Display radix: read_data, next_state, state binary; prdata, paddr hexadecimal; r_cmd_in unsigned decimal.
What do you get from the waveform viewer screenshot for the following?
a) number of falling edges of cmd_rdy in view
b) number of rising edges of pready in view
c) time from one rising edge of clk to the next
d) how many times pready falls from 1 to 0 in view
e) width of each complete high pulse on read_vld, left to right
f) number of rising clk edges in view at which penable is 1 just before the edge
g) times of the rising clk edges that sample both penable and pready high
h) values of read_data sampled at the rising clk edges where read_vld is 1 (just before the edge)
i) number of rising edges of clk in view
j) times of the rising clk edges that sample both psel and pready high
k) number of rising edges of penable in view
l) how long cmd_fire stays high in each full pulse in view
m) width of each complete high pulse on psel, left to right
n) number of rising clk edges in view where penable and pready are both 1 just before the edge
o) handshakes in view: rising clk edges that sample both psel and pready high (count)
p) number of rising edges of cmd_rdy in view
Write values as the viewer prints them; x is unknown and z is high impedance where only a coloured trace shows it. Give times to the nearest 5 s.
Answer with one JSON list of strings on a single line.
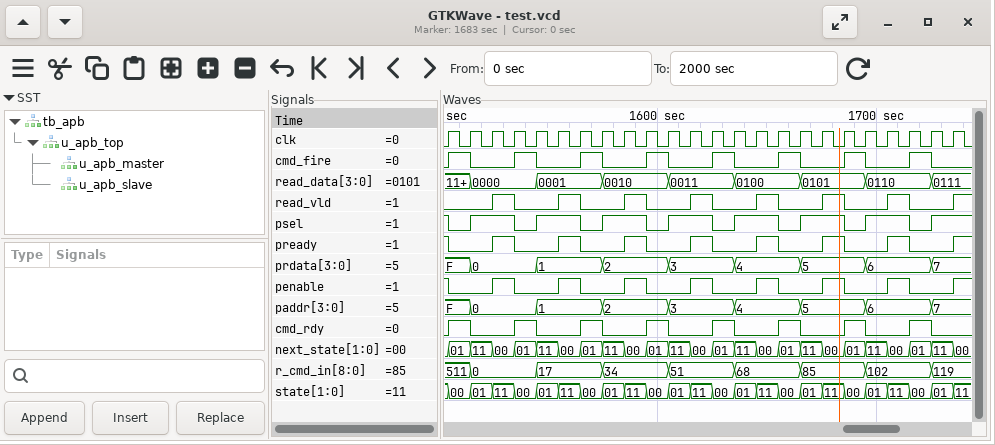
["8", "8", "10 s", "8", "10 s, 10 s, 10 s, 10 s, 10 s, 10 s, 10 s", "8", "1505 s, 1535 s, 1565 s, 1595 s, 1625 s, 1655 s, 1685 s, 1715 s", "0000, 0001, 0010, 0011, 0100, 0101, 0110", "24", "1505 s, 1535 s, 1565 s, 1595 s, 1625 s, 1655 s, 1685 s, 1715 s", "8", "10 s, 10 s, 10 s, 10 s, 10 s, 10 s, 10 s, 10 s", "20 s, 20 s, 20 s, 20 s, 20 s, 20 s, 20 s", "8", "8", "8"]
